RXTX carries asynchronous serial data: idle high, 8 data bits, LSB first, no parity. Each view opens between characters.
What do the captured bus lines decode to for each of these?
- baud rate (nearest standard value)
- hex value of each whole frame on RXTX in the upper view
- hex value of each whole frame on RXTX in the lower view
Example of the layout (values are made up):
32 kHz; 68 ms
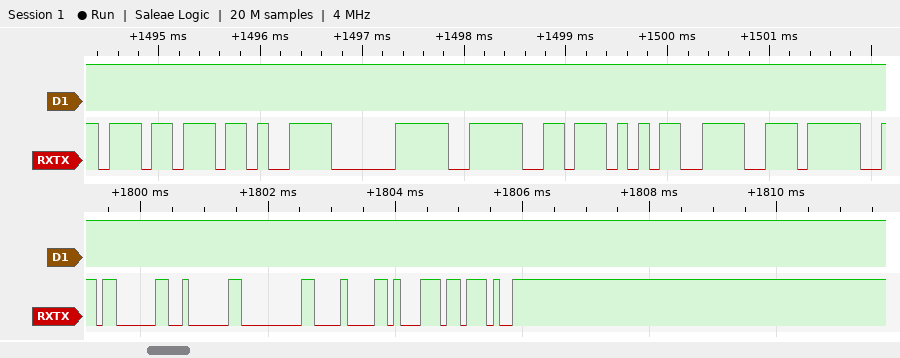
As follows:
9600 baud; B7, CB, E0, 3E, 57, 9E; 03, 02, 00, 08, 71, 97
